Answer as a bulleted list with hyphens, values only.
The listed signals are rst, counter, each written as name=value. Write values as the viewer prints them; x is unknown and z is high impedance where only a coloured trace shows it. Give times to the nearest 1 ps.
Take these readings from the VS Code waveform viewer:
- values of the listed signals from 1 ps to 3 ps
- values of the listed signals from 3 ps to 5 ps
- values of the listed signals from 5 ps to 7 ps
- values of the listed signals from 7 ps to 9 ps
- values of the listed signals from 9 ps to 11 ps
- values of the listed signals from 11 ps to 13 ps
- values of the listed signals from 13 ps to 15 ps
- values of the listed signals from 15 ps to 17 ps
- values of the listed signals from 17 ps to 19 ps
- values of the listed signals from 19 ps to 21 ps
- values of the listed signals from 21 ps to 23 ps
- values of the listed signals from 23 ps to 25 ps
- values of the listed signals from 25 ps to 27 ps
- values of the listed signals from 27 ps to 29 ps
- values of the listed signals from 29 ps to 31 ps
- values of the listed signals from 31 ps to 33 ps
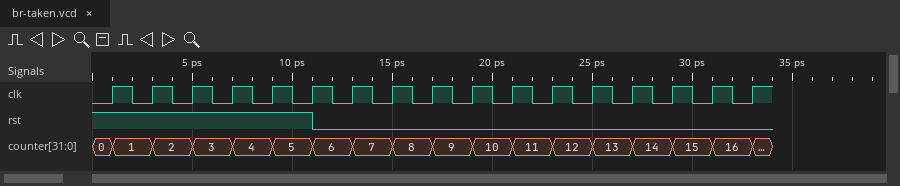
- rst=1, counter=1
- rst=1, counter=2
- rst=1, counter=3
- rst=1, counter=4
- rst=1, counter=5
- rst=0, counter=6
- rst=0, counter=7
- rst=0, counter=8
- rst=0, counter=9
- rst=0, counter=10
- rst=0, counter=11
- rst=0, counter=12
- rst=0, counter=13
- rst=0, counter=14
- rst=0, counter=15
- rst=0, counter=16
